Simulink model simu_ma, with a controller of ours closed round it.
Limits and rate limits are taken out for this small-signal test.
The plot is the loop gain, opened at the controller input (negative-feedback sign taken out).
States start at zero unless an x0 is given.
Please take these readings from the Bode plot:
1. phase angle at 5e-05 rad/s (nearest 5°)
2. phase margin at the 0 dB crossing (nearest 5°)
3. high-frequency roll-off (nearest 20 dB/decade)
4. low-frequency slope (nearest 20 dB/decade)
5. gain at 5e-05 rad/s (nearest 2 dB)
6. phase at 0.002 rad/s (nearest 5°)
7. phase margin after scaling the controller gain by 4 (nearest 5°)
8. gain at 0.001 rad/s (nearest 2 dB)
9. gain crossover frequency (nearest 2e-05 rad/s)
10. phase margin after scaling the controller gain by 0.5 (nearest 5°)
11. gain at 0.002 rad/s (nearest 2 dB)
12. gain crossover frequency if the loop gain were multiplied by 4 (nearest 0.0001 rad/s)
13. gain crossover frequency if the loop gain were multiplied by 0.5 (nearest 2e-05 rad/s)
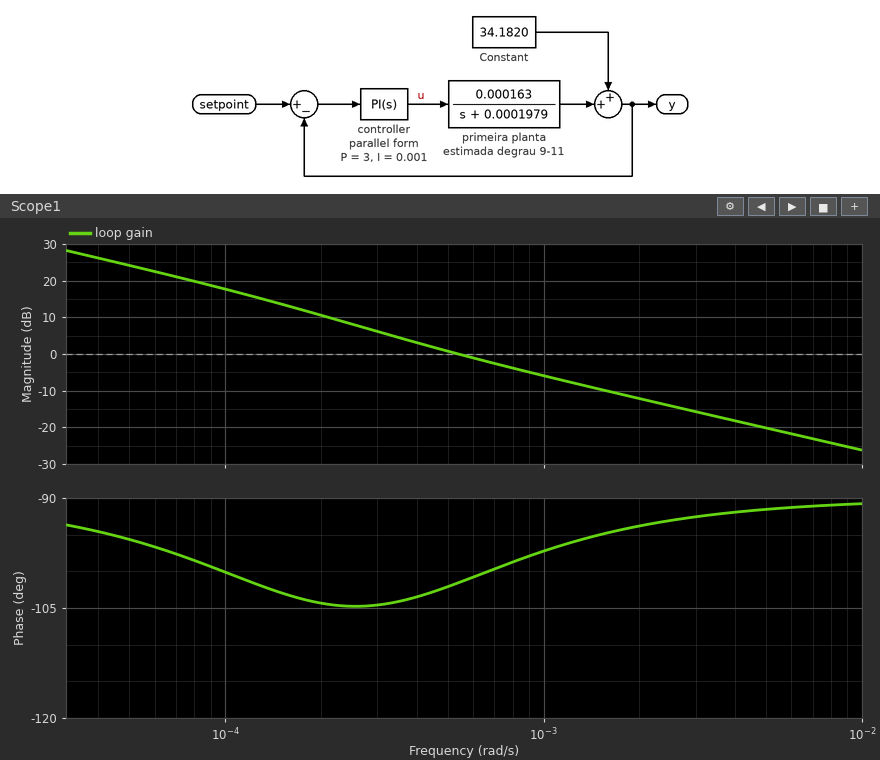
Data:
-95°
80°
-20 dB/decade
-20 dB/decade
24 dB
-95°
85°
-6 dB
0.00054 rad/s
75°
-12 dB
0.0020 rad/s
0.00030 rad/s
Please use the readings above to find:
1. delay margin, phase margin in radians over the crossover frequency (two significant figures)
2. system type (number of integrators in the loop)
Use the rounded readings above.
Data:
2600 s
1
